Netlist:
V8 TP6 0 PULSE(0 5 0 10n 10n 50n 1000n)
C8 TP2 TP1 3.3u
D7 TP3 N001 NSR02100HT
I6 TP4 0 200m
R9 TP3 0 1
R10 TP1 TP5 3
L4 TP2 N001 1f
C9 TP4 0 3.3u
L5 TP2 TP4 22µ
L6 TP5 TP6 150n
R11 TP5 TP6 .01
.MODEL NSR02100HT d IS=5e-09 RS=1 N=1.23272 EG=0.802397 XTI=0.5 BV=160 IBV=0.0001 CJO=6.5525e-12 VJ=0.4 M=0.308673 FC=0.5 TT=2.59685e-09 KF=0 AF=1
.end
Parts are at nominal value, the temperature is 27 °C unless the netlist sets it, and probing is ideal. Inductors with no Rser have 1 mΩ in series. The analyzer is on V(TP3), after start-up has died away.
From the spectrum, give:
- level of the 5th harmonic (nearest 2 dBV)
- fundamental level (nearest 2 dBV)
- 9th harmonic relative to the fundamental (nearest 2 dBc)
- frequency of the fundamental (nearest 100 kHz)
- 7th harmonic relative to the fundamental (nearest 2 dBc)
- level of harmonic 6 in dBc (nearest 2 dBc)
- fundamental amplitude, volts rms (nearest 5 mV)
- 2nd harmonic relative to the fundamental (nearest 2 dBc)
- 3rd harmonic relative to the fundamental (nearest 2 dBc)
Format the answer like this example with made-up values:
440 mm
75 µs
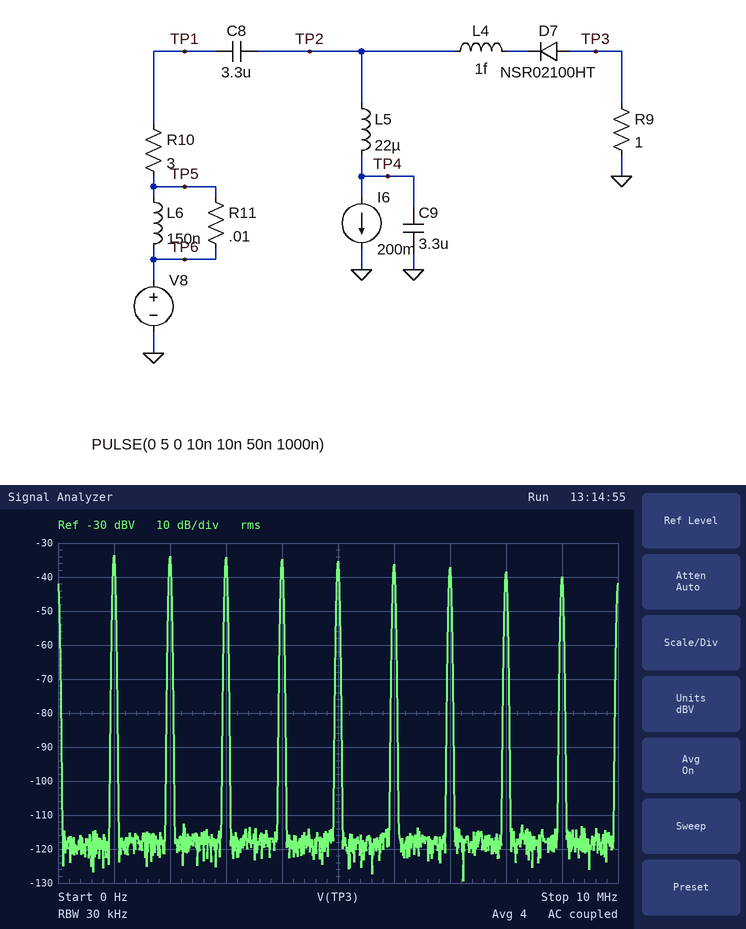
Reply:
-36 dBV
-34 dBV
-6 dBc
1.0 MHz
-4 dBc
-2 dBc
20 mV
0 dBc
0 dBc
